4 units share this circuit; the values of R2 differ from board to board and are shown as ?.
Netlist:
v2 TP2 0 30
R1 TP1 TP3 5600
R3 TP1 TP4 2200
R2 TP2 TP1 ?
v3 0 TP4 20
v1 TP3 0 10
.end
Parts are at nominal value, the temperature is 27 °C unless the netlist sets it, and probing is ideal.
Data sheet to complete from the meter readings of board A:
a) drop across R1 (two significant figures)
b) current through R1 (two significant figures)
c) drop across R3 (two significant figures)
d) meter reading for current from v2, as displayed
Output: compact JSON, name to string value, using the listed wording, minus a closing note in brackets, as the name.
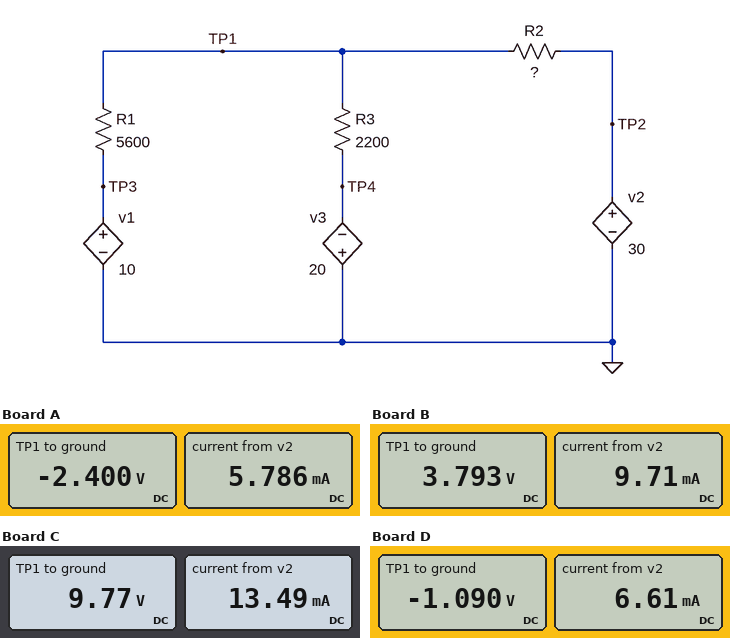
{"drop across R1": "12 V", "current through R1": "2.2 mA", "drop across R3": "18 V", "meter reading for current from v2, as displayed": "5.786 mA"}
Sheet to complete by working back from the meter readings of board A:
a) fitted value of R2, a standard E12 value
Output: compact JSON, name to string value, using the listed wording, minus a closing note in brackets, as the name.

{"fitted value of R2, a standard E12 value": "5.6 kΩ"}
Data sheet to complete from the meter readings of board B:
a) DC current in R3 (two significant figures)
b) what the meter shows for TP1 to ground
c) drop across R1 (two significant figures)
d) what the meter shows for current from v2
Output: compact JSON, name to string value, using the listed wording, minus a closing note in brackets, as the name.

{"DC current in R3": "11 mA", "what the meter shows for TP1 to ground": "3.793 V", "drop across R1": "6.2 V", "what the meter shows for current from v2": "9.71 mA"}
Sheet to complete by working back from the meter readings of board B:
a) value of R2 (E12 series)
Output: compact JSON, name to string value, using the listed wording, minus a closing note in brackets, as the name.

{"value of R2": "2.7 kΩ"}
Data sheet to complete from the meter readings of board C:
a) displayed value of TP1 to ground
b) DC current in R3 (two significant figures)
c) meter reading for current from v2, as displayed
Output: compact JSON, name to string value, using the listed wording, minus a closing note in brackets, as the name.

{"displayed value of TP1 to ground": "9.77 V", "DC current in R3": "14 mA", "meter reading for current from v2, as displayed": "13.49 mA"}
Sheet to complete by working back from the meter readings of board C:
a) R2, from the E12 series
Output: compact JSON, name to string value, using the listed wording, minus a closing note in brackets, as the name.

{"R2, from the E12 series": "1.5 kΩ"}
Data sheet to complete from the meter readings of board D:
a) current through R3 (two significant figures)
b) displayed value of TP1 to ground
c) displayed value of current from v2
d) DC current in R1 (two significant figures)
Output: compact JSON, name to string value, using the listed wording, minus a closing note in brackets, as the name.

{"current through R3": "8.6 mA", "displayed value of TP1 to ground": "-1.090 V", "displayed value of current from v2": "6.61 mA", "DC current in R1": "2.0 mA"}
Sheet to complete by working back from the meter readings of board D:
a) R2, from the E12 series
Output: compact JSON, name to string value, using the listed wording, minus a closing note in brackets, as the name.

{"R2, from the E12 series": "4.7 kΩ"}
